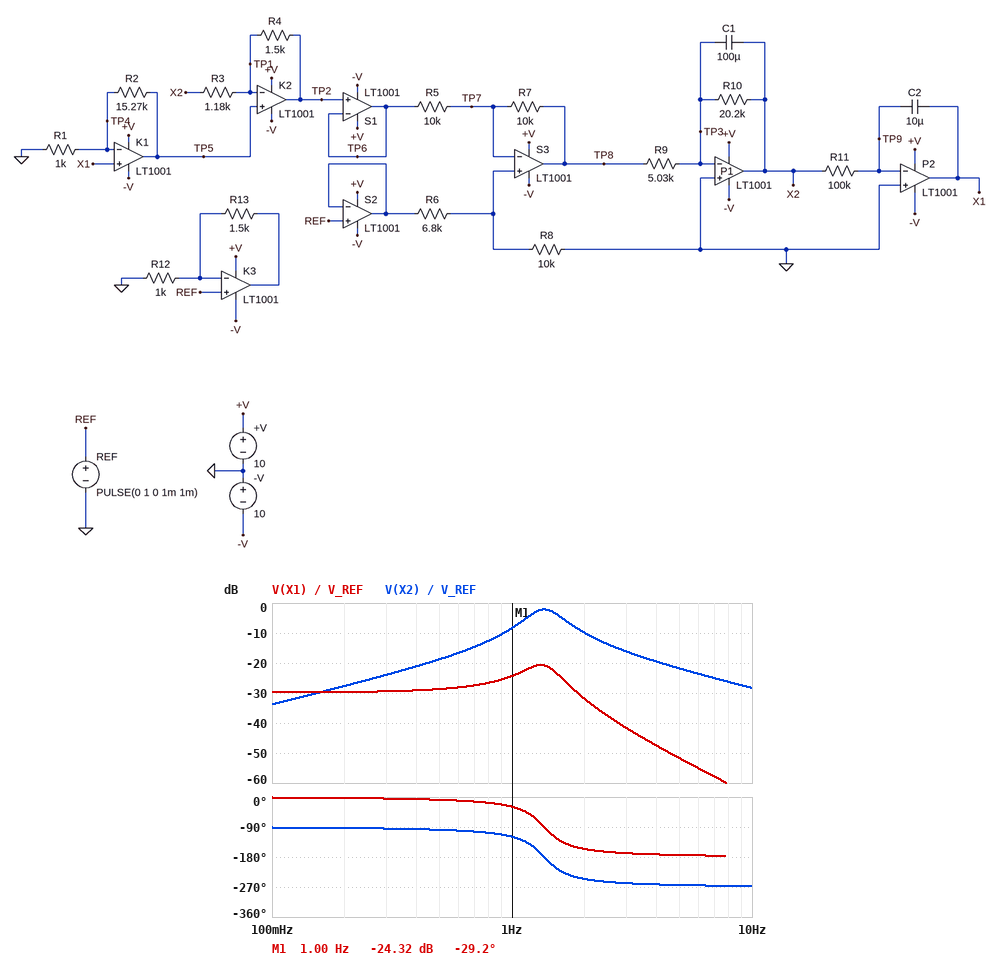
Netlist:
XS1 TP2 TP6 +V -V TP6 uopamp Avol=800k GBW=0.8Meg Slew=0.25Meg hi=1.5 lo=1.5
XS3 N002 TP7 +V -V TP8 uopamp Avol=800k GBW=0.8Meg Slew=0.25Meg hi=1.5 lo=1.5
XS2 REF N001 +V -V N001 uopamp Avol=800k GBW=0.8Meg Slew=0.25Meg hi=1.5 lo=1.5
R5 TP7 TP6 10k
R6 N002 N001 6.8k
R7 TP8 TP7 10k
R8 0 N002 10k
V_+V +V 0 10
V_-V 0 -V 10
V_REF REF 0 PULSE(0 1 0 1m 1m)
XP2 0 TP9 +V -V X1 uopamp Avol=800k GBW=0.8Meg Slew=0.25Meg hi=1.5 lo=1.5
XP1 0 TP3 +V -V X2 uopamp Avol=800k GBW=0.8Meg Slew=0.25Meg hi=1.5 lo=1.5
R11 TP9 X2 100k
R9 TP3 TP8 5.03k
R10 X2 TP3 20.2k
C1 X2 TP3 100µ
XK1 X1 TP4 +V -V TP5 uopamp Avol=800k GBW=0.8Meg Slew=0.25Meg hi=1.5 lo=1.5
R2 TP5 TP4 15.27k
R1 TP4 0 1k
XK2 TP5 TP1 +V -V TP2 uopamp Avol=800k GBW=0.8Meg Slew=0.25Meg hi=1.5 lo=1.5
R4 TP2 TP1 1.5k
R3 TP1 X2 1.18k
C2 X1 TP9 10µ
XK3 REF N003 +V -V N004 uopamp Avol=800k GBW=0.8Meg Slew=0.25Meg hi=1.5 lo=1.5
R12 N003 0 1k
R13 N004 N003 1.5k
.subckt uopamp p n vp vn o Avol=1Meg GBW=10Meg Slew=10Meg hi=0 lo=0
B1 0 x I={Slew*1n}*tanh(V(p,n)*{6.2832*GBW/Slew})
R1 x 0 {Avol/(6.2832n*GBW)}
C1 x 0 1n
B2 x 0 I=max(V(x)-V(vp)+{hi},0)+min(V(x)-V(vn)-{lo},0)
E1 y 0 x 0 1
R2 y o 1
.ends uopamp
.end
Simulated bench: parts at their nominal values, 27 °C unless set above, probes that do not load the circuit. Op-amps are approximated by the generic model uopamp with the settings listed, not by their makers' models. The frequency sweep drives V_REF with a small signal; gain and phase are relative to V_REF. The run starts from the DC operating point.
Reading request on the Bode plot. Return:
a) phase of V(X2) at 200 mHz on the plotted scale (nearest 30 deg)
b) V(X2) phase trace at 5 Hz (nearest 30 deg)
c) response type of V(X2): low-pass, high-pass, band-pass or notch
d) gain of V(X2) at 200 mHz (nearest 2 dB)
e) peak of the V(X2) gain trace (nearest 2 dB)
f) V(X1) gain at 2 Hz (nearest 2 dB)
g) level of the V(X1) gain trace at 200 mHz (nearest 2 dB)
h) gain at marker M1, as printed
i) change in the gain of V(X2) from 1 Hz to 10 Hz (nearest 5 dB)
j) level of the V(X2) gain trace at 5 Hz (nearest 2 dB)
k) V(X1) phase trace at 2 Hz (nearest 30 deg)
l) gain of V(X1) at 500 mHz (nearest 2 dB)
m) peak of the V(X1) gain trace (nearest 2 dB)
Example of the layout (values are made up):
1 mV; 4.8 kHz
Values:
-90 deg; -270 deg; band-pass; -28 dB; -2 dB; -32 dB; -30 dB; -24.32 dB; -20 dB; -22 dB; -150 deg; -28 dB; -20 dB
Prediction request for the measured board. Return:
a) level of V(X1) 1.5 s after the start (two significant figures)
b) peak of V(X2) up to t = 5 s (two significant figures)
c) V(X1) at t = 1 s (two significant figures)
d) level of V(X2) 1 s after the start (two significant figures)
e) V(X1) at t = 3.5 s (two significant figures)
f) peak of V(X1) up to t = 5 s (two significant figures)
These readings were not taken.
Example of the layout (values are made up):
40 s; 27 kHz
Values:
29 mV; 120 mV; 35 mV; -52 mV; 32 mV; 51 mV
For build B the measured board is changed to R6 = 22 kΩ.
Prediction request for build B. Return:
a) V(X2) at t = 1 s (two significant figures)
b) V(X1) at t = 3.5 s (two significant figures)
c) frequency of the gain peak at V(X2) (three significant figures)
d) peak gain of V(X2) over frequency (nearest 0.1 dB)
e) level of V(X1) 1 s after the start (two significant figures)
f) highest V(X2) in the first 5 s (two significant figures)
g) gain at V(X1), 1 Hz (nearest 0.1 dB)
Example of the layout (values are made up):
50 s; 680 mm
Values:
-27 mV; 17 mV; 1.36 Hz; -7.7 dB; 18 mV; 64 mV; -29.9 dB
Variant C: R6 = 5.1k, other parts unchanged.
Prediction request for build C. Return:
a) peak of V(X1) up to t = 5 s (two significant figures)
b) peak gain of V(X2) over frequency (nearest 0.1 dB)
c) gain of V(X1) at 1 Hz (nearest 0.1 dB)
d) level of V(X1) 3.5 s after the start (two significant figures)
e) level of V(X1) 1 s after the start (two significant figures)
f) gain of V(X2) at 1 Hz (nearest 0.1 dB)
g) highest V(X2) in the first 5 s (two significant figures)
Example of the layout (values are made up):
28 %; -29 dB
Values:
56 mV; -1.2 dB; -23.4 dB; 36 mV; 39 mV; -7.4 dB; 140 mV
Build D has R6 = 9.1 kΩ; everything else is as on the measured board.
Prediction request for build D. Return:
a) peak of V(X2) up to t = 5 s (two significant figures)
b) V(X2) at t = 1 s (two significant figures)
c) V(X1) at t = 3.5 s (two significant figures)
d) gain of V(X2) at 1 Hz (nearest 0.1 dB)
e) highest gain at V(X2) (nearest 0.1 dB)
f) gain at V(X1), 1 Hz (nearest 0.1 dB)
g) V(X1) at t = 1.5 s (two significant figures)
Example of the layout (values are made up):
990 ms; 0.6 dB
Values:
110 mV; -46 mV; 28 mV; -9.5 dB; -3.2 dB; -25.4 dB; 25 mV
